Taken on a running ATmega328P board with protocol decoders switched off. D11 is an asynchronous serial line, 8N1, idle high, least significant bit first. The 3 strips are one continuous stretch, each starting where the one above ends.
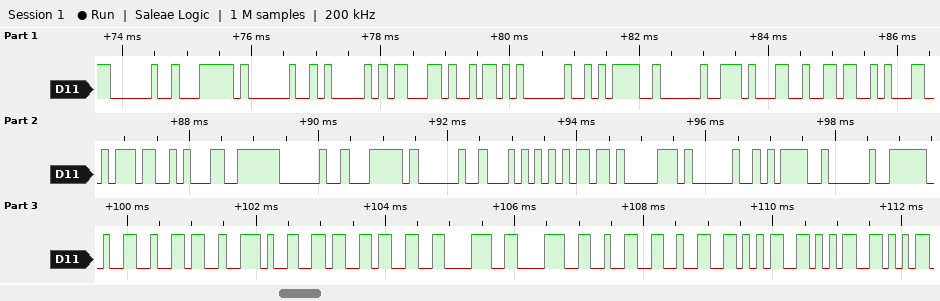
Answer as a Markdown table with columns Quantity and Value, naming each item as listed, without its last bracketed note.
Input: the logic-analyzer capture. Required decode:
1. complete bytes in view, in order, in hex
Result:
| Quantity | Value |
|---|---|
| complete bytes in view, in order, in hex | 20 7C 20 41 63 5A 20 3D 20 31 36 31 37 31 20 7C 20 54 6D 70 20 3D 20 32 36 2E 36 33 38 38 32 32 35 35 |
